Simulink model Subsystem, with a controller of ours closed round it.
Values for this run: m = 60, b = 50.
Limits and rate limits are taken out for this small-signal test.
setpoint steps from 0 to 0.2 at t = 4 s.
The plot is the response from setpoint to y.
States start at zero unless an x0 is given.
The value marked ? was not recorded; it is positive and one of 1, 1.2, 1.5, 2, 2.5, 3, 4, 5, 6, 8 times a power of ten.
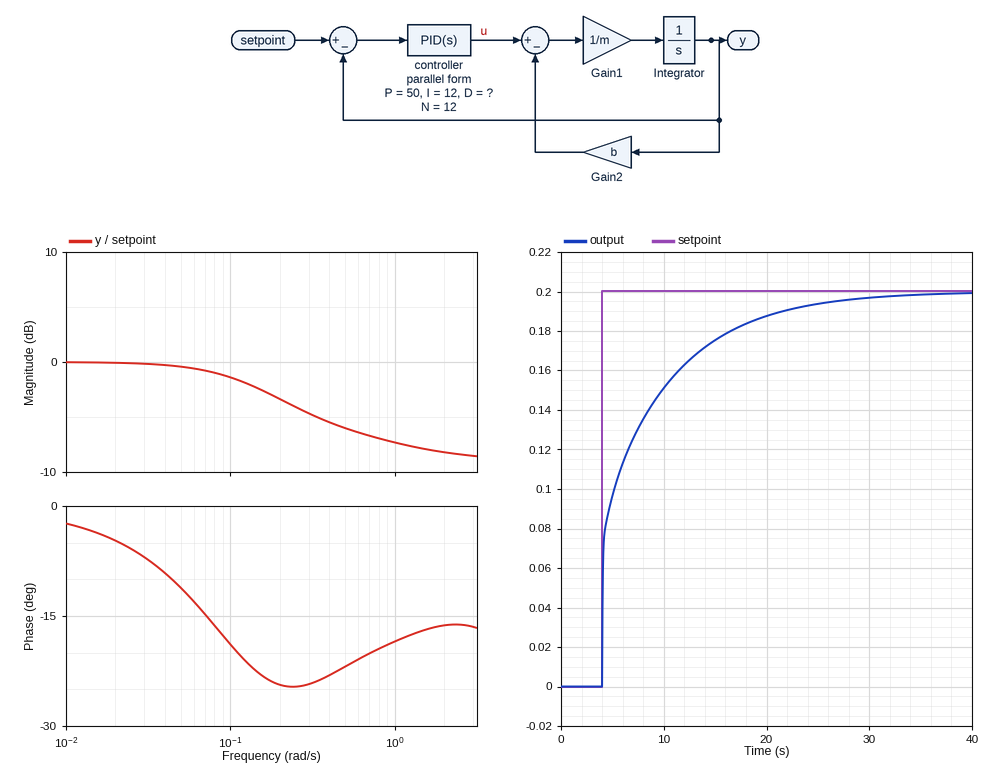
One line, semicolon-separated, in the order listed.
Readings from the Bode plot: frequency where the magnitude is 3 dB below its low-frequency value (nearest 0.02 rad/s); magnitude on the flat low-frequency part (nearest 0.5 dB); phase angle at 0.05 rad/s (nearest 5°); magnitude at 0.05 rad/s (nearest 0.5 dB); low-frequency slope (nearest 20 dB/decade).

0.18 rad/s; 0.0 dB; -10°; -0.5 dB; 0 dB/decade
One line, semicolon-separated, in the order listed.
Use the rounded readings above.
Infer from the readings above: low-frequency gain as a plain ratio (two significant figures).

1.0
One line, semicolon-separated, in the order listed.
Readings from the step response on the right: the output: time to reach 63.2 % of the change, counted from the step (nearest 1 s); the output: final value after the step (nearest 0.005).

3 s; 0.200
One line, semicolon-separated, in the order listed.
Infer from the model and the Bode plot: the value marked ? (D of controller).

30
